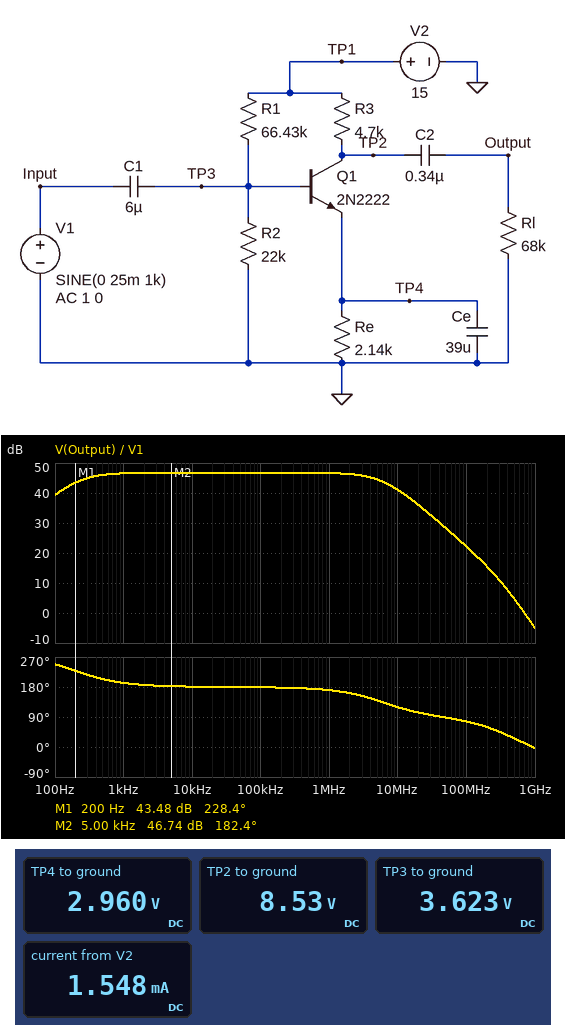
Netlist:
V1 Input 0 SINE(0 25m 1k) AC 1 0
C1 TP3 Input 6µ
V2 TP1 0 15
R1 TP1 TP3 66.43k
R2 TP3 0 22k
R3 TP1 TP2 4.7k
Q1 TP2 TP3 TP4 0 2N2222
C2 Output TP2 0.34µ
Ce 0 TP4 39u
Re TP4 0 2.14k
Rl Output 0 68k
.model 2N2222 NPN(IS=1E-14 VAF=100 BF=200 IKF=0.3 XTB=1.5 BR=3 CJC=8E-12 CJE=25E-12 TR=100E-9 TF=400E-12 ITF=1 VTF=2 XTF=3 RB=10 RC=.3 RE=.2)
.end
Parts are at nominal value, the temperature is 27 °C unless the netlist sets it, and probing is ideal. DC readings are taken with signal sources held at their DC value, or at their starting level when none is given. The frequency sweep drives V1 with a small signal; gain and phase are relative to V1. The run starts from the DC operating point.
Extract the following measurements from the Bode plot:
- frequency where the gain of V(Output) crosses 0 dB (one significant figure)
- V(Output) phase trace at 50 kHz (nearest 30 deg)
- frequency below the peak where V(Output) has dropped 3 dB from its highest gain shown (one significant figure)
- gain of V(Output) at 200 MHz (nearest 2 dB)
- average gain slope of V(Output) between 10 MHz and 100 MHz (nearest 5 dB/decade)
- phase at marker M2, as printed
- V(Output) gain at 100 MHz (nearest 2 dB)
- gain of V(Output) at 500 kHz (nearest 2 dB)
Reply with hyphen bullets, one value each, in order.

- 700 MHz
- 180 deg
- 200 Hz
- 16 dB
- -20 dB/decade
- 182.4 deg
- 22 dB
- 46 dB
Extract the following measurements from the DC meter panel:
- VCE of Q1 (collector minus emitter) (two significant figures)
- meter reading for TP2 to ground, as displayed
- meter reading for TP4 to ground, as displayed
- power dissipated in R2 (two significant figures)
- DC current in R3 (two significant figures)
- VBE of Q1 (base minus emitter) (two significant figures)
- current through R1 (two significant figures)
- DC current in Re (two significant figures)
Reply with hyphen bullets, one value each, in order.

- 5.6 V
- 8.53 V
- 2.960 V
- 600 µW
- 1.4 mA
- 660 mV
- 170 µA
- 1.4 mA
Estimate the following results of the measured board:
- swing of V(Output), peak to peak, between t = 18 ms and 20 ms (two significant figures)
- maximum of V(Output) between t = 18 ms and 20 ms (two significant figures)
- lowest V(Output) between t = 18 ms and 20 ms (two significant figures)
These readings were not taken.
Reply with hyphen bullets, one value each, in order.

- 9.5 V
- 4.0 V
- -5.5 V
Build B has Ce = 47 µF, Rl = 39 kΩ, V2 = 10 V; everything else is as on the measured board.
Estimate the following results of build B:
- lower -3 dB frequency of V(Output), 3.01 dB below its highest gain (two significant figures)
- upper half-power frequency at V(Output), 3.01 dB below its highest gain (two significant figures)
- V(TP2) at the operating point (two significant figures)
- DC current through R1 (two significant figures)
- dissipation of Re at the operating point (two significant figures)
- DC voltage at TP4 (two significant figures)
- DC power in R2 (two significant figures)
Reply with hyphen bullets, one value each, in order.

- 110 Hz
- 6.7 MHz
- 6.1 V
- 110 µA
- 1.5 mW
- 1.8 V
- 270 µW
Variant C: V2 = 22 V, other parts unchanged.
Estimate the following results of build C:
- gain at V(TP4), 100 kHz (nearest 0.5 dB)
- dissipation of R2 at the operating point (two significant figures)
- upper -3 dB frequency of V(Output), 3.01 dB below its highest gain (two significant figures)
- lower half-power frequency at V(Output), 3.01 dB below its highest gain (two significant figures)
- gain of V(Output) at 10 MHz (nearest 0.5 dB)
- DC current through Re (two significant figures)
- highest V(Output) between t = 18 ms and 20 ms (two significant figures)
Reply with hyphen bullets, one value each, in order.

- -50.5 dB
- 1.3 mW
- 5.7 MHz
- 320 Hz
- 44.0 dB
- 2.2 mA
- 6.0 V
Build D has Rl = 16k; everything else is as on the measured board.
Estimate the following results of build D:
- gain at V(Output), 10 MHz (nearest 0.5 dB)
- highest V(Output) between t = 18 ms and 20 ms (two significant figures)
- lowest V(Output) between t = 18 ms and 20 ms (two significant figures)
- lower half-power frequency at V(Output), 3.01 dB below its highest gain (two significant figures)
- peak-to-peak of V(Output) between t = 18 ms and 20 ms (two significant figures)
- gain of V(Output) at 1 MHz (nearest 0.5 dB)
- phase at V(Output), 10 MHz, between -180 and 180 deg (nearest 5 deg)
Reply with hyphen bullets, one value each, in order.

- 40.5 dB
- 3.3 V
- -5.0 V
- 220 Hz
- 8.3 V
- 45.0 dB
- 125 deg
